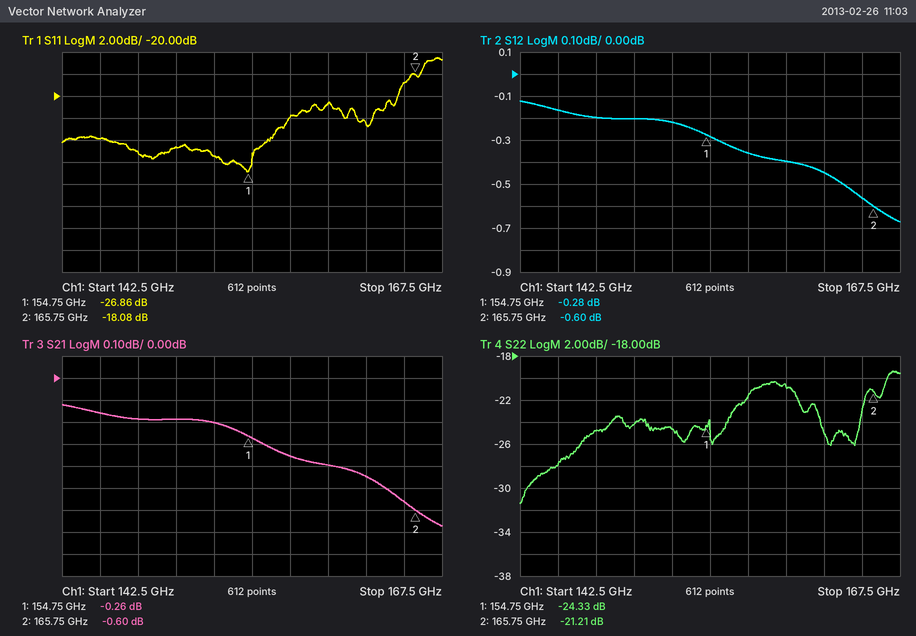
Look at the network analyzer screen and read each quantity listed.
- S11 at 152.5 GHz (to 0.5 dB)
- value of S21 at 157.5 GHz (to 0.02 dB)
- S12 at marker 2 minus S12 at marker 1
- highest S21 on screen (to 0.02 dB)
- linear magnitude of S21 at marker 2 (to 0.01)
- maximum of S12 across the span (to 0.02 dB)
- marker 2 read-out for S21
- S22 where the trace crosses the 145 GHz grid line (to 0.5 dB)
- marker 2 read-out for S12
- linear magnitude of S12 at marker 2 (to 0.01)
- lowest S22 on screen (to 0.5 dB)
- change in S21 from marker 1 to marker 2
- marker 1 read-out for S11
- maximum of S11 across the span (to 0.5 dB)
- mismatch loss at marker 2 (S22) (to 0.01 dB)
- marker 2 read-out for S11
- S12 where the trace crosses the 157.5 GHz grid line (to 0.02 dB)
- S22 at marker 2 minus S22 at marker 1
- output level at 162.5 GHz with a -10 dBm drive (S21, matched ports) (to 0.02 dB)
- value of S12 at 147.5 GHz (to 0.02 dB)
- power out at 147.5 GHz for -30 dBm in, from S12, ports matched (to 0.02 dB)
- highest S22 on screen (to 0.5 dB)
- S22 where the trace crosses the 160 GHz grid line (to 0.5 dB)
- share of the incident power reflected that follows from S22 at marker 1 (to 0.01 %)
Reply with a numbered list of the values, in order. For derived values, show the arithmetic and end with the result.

1. -25.5 dB
2. -0.36 dB
3. -0.6 − (-0.28) = -0.32 dB
4. -0.12 dB
5. 10^(-0.6/20) ≈ 0.93
6. -0.12 dB
7. -0.60 dB
8. -28.0 dB
9. -0.60 dB
10. 10^(-0.6/20) ≈ 0.93
11. -31.5 dB
12. -0.6 − (-0.26) = -0.34 dB
13. -26.86 dB
14. -16.5 dB
15. −10 log10(1 − 10^(-21.21/10)) ≈ 0.03 dB
16. -18.08 dB
17. -0.36 dB
18. -21.21 − (-24.33) = 3.12 dB
19. -10 dBm + (-0.44 dB) = -10.44 dBm
20. -0.20 dB
21. -30 dBm + (-0.20 dB) = -30.20 dBm
22. -19.5 dB
23. -21.0 dB
24. 10^(-24.33/10) ≈ 0.37 %
